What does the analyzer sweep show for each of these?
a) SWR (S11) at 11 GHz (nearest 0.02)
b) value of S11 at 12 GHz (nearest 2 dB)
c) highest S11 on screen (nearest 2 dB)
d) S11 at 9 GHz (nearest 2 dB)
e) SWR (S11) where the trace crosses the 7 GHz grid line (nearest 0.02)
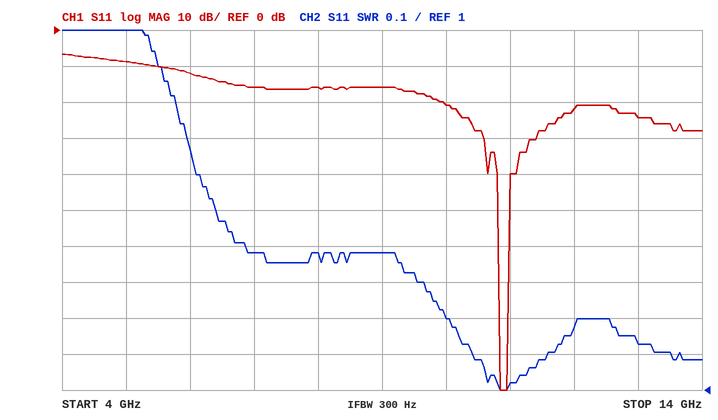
1.02
-22 dB
-6 dB
-16 dB
1.38
